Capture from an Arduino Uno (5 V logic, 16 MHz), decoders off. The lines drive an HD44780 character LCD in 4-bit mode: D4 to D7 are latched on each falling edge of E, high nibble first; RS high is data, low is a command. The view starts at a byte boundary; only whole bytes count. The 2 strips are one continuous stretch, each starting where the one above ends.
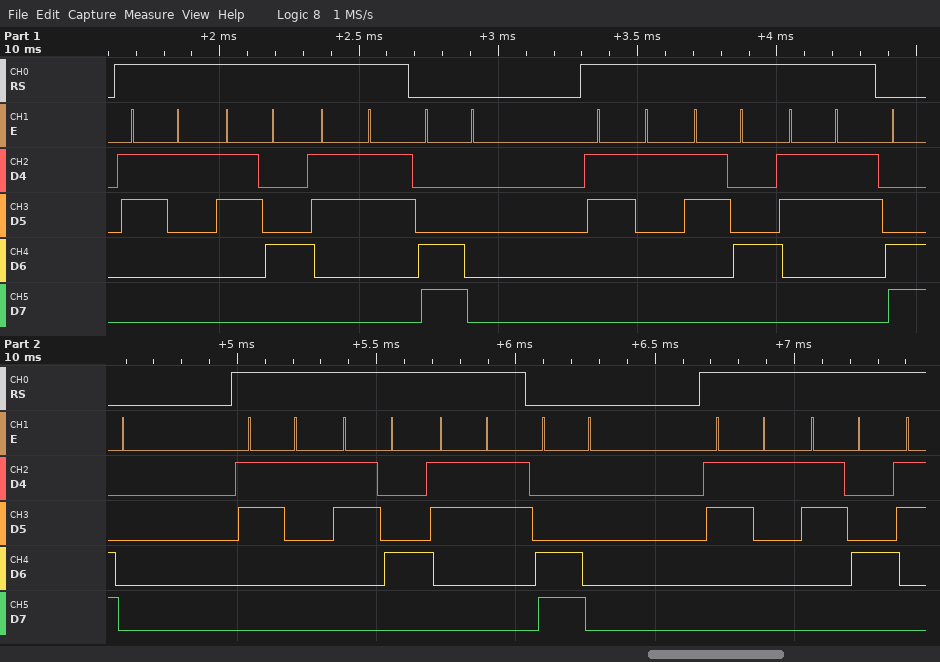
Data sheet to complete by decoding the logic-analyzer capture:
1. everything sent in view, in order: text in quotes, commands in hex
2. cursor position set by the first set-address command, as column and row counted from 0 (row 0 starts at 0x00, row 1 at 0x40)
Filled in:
"143" 0xC0 "143" 0xC0 "143" 0xC0 "14"
column 0, row 1
